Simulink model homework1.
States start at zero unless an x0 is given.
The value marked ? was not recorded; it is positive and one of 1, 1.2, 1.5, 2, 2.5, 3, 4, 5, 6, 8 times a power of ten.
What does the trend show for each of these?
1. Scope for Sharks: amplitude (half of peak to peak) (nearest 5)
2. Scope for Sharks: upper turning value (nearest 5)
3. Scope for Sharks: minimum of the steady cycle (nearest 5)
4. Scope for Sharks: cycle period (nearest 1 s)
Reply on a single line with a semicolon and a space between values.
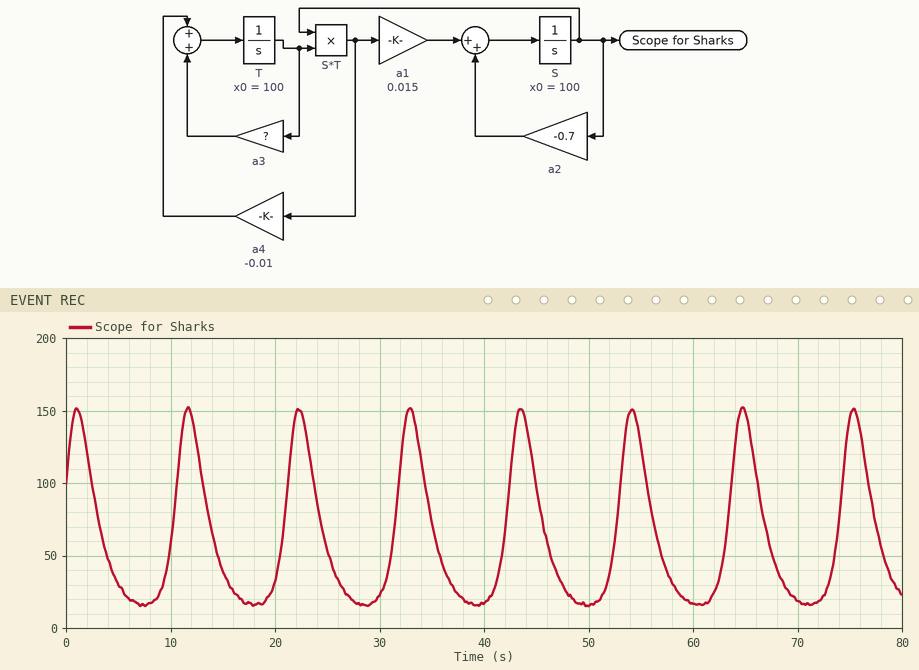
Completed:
70; 150; 15; 11 s
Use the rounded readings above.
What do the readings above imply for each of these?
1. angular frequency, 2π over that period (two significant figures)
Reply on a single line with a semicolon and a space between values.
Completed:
0.57 rad/s
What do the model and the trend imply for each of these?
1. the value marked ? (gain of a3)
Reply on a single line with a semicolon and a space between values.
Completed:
0.6
